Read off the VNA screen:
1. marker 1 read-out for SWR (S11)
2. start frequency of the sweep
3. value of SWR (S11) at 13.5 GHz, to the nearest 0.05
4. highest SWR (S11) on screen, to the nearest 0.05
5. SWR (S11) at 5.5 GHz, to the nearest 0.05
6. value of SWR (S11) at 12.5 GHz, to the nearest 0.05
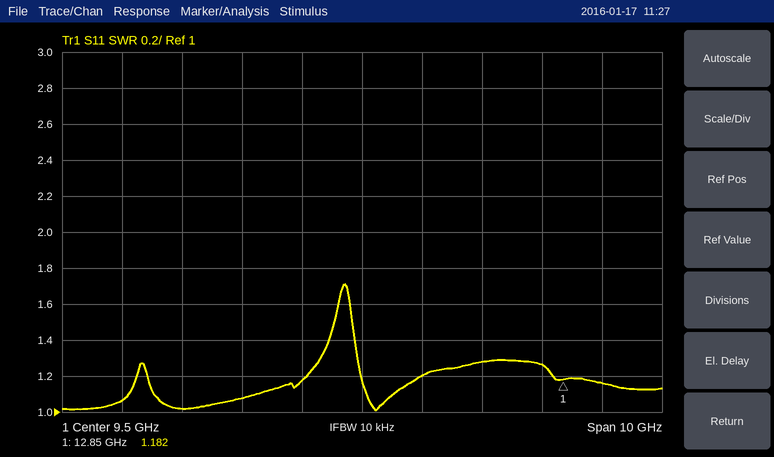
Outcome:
1.182
4.5 GHz
1.15
1.70
1.05
1.25
